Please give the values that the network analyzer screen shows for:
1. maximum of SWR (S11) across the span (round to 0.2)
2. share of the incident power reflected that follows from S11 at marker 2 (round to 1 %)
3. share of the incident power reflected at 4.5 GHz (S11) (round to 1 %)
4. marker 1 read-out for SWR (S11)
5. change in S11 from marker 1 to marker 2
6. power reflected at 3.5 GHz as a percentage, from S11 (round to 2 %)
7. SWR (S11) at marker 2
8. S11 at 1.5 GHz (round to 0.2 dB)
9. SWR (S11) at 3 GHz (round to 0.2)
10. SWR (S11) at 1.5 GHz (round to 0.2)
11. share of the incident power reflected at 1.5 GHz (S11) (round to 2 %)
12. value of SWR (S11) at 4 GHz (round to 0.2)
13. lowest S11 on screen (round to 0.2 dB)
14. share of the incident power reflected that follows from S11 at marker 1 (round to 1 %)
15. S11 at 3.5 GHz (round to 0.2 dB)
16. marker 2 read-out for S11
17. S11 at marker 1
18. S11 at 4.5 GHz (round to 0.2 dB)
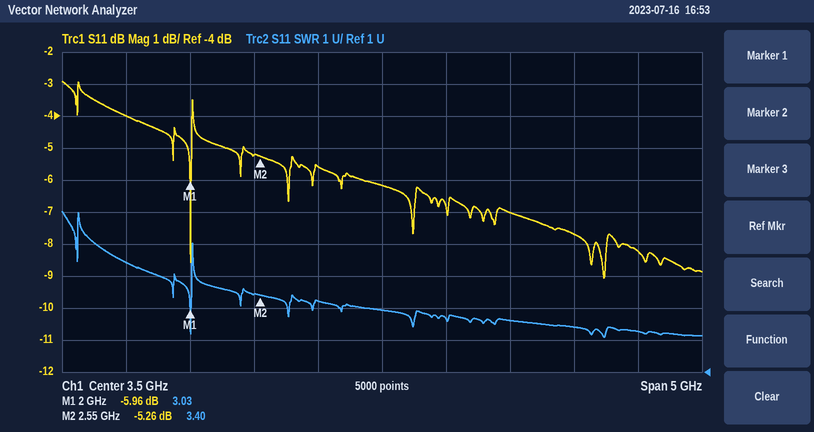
6.0
30 %
20 %
3.03
0.70 dB
24 %
3.40
-4.0 dB
3.2
4.4
40 %
2.6
-9.0 dB
25 %
-6.2 dB
-5.26 dB
-5.96 dB
-7.0 dB
